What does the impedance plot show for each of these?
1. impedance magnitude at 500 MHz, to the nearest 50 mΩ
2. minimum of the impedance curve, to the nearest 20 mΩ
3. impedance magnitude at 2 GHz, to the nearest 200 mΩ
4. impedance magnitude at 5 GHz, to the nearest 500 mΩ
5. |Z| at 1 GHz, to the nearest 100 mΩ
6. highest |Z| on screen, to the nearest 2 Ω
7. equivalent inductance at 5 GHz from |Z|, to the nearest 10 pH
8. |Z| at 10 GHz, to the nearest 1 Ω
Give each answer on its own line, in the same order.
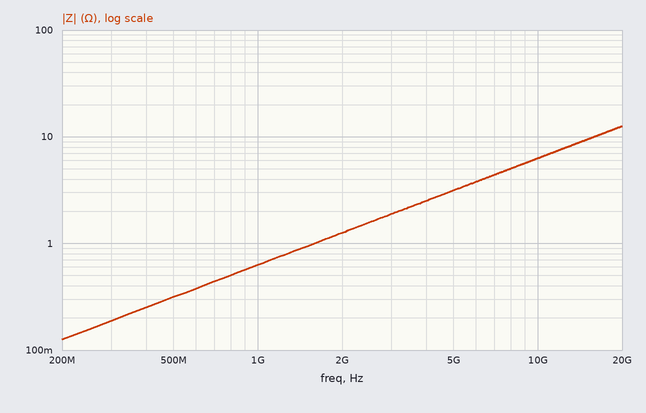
300 mΩ
120 mΩ
1.2 Ω
3.0 Ω
600 mΩ
12 Ω
100 pH
6 Ω
